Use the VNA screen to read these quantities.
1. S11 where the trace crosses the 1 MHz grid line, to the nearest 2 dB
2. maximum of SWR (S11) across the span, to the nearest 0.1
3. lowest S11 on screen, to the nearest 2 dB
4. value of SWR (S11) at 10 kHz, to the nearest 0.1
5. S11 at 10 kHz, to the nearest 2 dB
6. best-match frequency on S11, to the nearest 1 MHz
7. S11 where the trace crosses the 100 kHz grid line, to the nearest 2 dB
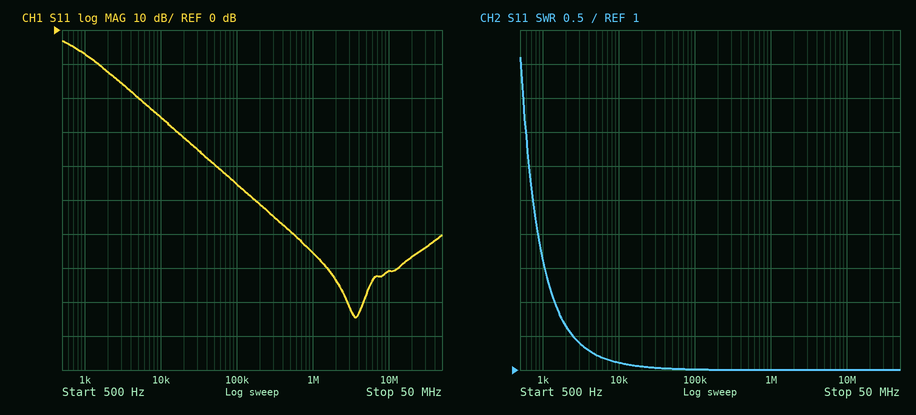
-66 dB
5.6
-84 dB
1.1
-26 dB
4 MHz
-46 dB
